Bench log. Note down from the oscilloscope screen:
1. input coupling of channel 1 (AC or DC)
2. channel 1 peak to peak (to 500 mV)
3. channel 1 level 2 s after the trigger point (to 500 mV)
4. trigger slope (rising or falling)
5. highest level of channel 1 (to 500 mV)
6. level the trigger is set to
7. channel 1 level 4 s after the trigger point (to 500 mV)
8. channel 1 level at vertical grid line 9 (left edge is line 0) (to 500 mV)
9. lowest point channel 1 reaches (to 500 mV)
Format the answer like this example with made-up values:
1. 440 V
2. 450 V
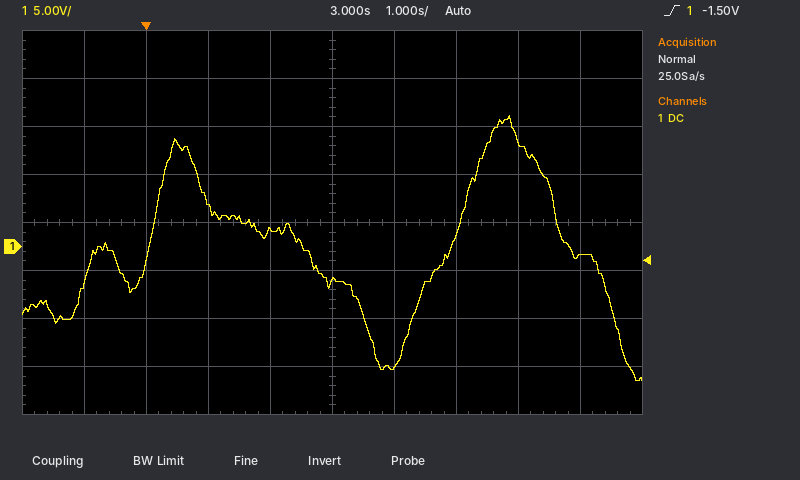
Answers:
1. DC
2. 27.5 V
3. 1.5 V
4. rising
5. 13.5 V
6. -1.50 V
7. -12.5 V
8. -1.0 V
9. -14.0 V
